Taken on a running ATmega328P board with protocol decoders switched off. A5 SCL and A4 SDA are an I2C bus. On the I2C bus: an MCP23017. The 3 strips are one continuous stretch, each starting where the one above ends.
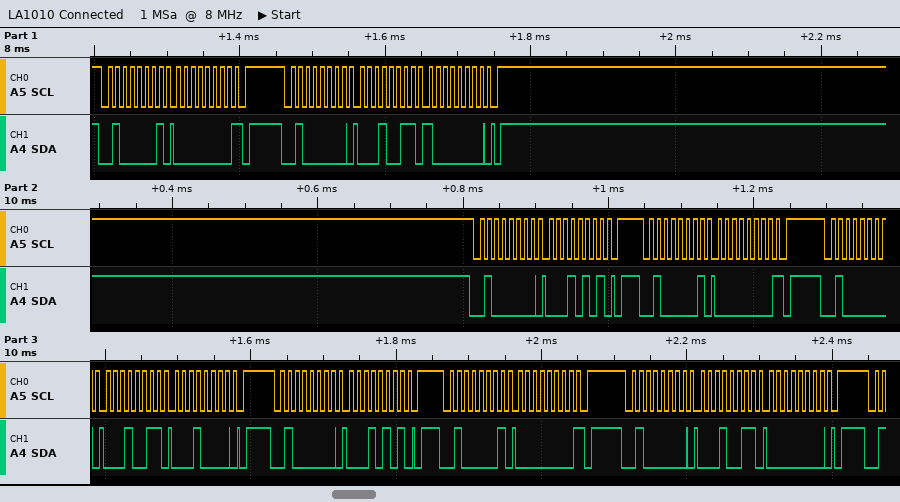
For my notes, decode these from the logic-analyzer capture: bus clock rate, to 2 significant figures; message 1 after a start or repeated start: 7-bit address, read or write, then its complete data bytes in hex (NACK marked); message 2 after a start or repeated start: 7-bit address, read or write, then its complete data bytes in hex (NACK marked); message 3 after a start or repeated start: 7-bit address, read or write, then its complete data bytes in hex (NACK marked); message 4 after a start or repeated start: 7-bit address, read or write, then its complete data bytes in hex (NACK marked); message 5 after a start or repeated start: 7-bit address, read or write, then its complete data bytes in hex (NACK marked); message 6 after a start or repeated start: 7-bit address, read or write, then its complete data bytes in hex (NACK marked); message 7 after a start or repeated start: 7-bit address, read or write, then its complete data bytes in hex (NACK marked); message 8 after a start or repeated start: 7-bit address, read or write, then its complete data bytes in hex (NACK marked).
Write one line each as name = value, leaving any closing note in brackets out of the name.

bus clock rate, to 2 significant figures = 100 kHz
message 1 after a start or repeated start: 7-bit address, read or write, then its complete data bytes in hex = 0x20 read: 00 NACK
message 2 after a start or repeated start: 7-bit address, read or write, then its complete data bytes in hex = 0x20 write: 13 80
message 3 after a start or repeated start: 7-bit address, read or write, then its complete data bytes in hex = 0x20 write: 15
message 4 after a start or repeated start: 7-bit address, read or write, then its complete data bytes in hex = 0x20 read: 00 NACK
message 5 after a start or repeated start: 7-bit address, read or write, then its complete data bytes in hex = 0x20 write: 13 10
message 6 after a start or repeated start: 7-bit address, read or write, then its complete data bytes in hex = 0x20 write: 15
message 7 after a start or repeated start: 7-bit address, read or write, then its complete data bytes in hex = 0x20 read: 00 NACK
message 8 after a start or repeated start: 7-bit address, read or write, then its complete data bytes in hex = 0x20 write: 13 00
